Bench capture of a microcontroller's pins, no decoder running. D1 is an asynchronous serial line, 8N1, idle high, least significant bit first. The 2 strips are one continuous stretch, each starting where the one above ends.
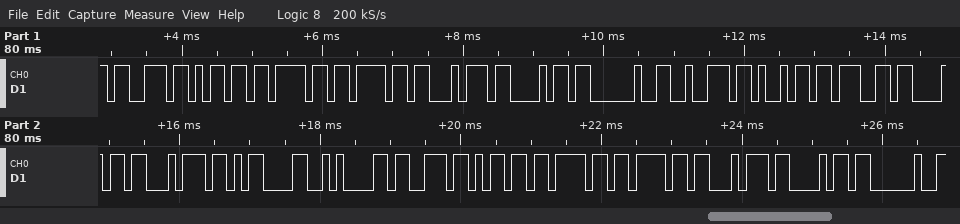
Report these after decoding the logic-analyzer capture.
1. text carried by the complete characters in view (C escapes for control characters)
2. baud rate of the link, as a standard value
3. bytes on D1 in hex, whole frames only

"smooth right\r\nsmooth "
9600 baud
0x73 0x6D 0x6F 0x6F 0x74 0x68 0x20 0x72 0x69 0x67 0x68 0x74 0x0D 0x0A 0x73 0x6D 0x6F 0x6F 0x74 0x68 0x20
